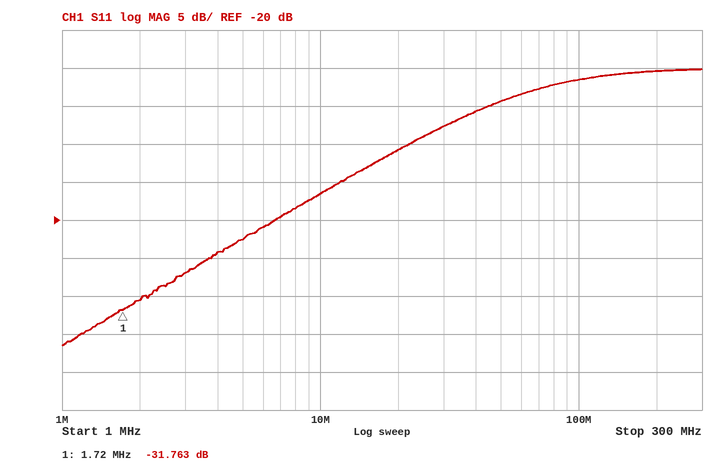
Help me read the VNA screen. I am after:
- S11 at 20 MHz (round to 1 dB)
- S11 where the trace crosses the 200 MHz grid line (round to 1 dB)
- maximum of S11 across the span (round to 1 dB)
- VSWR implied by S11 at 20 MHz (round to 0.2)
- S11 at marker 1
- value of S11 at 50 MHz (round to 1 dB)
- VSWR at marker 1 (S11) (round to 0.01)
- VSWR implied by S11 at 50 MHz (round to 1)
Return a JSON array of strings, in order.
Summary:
["-11 dB", "0 dB", "0 dB", "1.8", "-31.763 dB", "-4 dB", "1.05", "4"]
